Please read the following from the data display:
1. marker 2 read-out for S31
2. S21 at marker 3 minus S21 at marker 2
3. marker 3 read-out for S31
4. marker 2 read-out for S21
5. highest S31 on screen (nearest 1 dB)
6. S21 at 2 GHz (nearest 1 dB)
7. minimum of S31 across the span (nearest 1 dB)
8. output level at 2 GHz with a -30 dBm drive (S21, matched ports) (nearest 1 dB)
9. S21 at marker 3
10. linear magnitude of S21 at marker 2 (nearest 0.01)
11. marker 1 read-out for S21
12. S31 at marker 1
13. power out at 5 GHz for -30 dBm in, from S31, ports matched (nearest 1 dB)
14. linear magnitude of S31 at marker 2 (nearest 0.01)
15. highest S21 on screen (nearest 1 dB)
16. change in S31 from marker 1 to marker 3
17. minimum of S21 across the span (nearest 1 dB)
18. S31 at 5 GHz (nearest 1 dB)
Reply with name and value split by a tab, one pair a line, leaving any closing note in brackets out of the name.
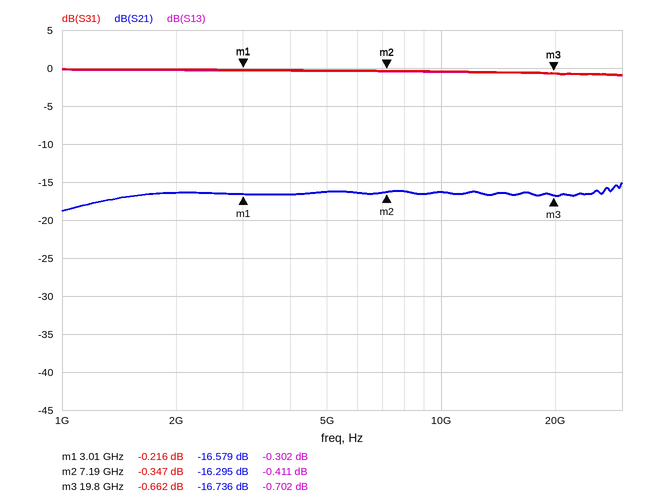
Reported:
marker 2 read-out for S31	-0.347 dB
S21 at marker 3 minus S21 at marker 2	-0.441 dB
marker 3 read-out for S31	-0.662 dB
marker 2 read-out for S21	-16.295 dB
highest S31 on screen	0 dB
S21 at 2 GHz	-16 dB
minimum of S31 across the span	-1 dB
output level at 2 GHz with a -30 dBm drive (S21, matched ports)	-46 dBm
S21 at marker 3	-16.736 dB
linear magnitude of S21 at marker 2	0.15
marker 1 read-out for S21	-16.579 dB
S31 at marker 1	-0.216 dB
power out at 5 GHz for -30 dBm in, from S31, ports matched	-30 dBm
linear magnitude of S31 at marker 2	0.96
highest S21 on screen	-15 dB
change in S31 from marker 1 to marker 3	-0.446 dB
minimum of S21 across the span	-19 dB
S31 at 5 GHz	0 dB
